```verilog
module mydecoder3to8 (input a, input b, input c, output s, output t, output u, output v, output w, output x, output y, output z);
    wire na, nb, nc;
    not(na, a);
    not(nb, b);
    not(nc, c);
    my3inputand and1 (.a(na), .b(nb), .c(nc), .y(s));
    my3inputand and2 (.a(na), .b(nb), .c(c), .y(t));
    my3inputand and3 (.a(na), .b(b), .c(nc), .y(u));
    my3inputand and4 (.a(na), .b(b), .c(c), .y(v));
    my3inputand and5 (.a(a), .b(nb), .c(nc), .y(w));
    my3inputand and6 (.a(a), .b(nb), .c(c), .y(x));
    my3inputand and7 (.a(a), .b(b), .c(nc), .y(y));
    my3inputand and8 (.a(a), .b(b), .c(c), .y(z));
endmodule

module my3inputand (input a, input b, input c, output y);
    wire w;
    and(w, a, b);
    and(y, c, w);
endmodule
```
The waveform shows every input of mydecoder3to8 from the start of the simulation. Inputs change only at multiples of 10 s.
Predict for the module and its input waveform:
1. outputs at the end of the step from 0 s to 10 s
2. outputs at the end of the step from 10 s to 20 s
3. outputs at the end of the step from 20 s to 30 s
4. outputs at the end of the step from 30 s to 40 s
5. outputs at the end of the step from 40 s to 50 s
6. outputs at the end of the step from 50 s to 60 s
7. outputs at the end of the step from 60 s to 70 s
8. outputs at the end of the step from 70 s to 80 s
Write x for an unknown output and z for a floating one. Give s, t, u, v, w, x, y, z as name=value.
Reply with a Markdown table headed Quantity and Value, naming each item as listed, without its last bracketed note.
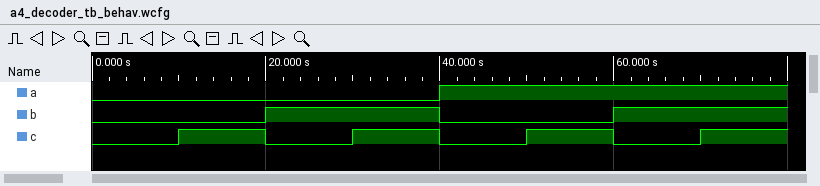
| Quantity | Value |
|---|---|
| outputs at the end of the step from 0 s to 10 s | s=1, t=0, u=0, v=0, w=0, x=0, y=0, z=0 |
| outputs at the end of the step from 10 s to 20 s | s=0, t=1, u=0, v=0, w=0, x=0, y=0, z=0 |
| outputs at the end of the step from 20 s to 30 s | s=0, t=0, u=1, v=0, w=0, x=0, y=0, z=0 |
| outputs at the end of the step from 30 s to 40 s | s=0, t=0, u=0, v=1, w=0, x=0, y=0, z=0 |
| outputs at the end of the step from 40 s to 50 s | s=0, t=0, u=0, v=0, w=1, x=0, y=0, z=0 |
| outputs at the end of the step from 50 s to 60 s | s=0, t=0, u=0, v=0, w=0, x=1, y=0, z=0 |
| outputs at the end of the step from 60 s to 70 s | s=0, t=0, u=0, v=0, w=0, x=0, y=1, z=0 |
| outputs at the end of the step from 70 s to 80 s | s=0, t=0, u=0, v=0, w=0, x=0, y=0, z=1 |
